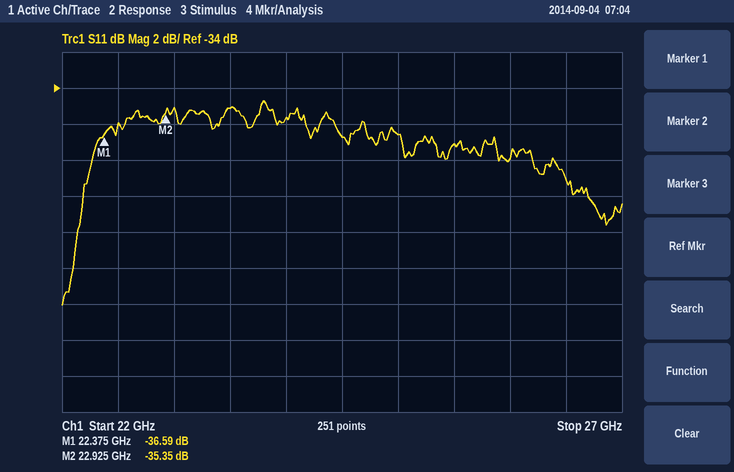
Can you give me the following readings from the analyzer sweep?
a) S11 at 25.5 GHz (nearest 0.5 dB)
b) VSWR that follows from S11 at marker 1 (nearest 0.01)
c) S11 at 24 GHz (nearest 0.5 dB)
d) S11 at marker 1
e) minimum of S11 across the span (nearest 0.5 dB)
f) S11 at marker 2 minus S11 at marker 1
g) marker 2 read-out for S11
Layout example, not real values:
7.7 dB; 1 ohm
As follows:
-37.0 dB; 1.03; -35.5 dB; -36.59 dB; -46.0 dB; 1.24 dB; -35.35 dB
